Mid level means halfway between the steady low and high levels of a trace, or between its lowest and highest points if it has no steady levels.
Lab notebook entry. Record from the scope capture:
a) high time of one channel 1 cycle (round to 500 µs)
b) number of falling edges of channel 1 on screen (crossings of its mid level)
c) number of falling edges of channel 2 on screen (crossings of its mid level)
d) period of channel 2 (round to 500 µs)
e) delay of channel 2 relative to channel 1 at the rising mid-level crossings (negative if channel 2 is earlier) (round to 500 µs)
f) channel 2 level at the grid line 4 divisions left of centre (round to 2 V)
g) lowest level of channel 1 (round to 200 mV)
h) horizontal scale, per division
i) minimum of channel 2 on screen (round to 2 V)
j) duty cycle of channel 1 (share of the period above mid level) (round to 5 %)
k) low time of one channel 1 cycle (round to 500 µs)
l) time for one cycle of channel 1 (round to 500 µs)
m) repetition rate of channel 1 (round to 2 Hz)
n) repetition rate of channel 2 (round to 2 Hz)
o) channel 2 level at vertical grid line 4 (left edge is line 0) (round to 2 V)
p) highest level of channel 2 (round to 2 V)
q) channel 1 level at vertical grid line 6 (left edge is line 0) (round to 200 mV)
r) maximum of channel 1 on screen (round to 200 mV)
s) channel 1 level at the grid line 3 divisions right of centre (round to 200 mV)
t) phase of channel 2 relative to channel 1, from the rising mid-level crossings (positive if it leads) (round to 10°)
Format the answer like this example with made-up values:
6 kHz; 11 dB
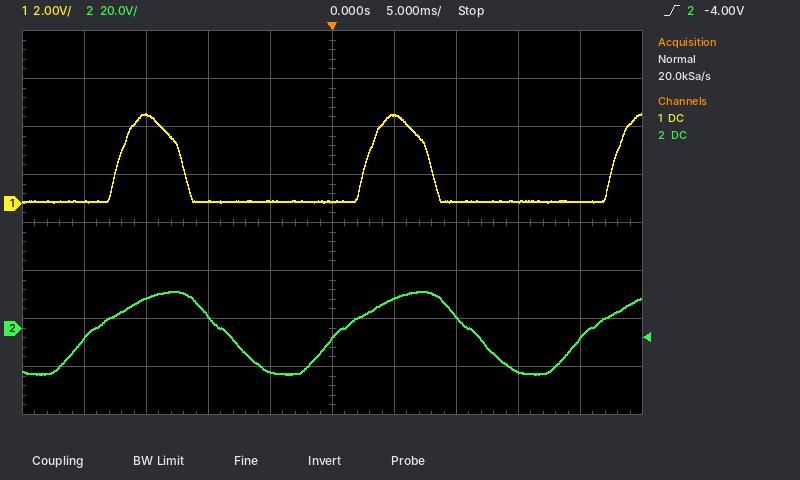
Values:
5.0 ms; 2; 2; 20.0 ms; -2.5 ms; -4 V; 0.0 V; 5 ms; -20 V; 25 %; 15.0 ms; 20.0 ms; 50 Hz; 50 Hz; -18 V; 16 V; 3.6 V; 3.8 V; 0.0 V; +40°
